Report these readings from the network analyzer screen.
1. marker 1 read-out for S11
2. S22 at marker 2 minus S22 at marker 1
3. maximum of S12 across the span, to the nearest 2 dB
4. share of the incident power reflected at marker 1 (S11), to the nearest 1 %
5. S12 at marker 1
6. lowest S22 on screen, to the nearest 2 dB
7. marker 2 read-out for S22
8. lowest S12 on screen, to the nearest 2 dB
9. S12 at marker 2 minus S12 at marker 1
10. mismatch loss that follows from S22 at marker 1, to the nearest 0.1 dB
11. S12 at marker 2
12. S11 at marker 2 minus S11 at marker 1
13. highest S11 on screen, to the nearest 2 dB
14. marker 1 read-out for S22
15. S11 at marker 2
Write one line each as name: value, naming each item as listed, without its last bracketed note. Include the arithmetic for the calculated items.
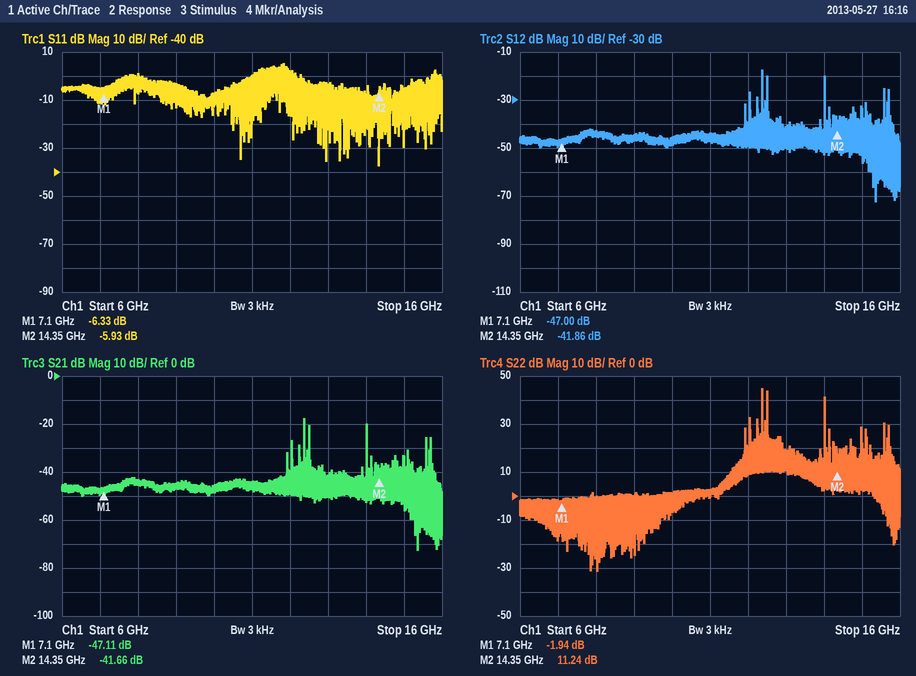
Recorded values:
marker 1 read-out for S11: -6.33 dB
S22 at marker 2 minus S22 at marker 1: 11.24 − (-1.94) = 13.18 dB
maximum of S12 across the span, to the nearest 2 dB: -18 dB
share of the incident power reflected at marker 1 (S11), to the nearest 1 %: 10^(-6.33/10) ≈ 23 %
S12 at marker 1: -47.00 dB
lowest S22 on screen, to the nearest 2 dB: -32 dB
marker 2 read-out for S22: 11.24 dB
lowest S12 on screen, to the nearest 2 dB: -72 dB
S12 at marker 2 minus S12 at marker 1: -41.86 − (-47) = 5.14 dB
mismatch loss that follows from S22 at marker 1, to the nearest 0.1 dB: −10 log10(1 − 10^(-1.94/10)) ≈ 4.4 dB
S12 at marker 2: -41.86 dB
S11 at marker 2 minus S11 at marker 1: -5.93 − (-6.33) = 0.40 dB
highest S11 on screen, to the nearest 2 dB: 6 dB
marker 1 read-out for S22: -1.94 dB
S11 at marker 2: -5.93 dB
